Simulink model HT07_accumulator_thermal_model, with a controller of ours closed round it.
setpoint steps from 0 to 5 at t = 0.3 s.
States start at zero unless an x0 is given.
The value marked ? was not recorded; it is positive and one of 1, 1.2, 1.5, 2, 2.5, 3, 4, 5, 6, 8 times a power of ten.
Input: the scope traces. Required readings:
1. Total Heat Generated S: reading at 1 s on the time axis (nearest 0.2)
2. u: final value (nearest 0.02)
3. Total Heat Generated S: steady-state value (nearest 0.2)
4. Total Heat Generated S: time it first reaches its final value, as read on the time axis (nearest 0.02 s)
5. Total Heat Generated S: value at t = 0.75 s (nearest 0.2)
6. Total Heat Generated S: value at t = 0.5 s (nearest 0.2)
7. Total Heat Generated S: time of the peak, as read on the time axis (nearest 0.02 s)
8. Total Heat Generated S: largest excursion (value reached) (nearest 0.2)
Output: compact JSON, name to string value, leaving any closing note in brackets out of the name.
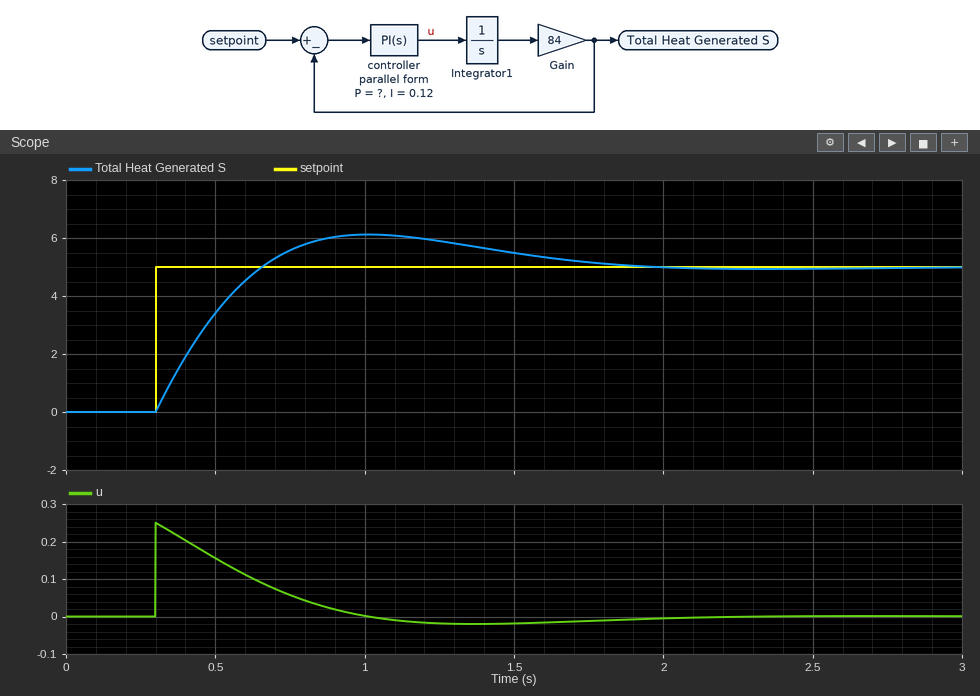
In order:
{"Total Heat Generated S: reading at 1 s on the time axis": "6.2", "u: final value": "0.00", "Total Heat Generated S: steady-state value": "5.0", "Total Heat Generated S: time it first reaches its final value, as read on the time axis": "0.66 s", "Total Heat Generated S: value at t = 0.75 s": "5.6", "Total Heat Generated S: value at t = 0.5 s": "3.4", "Total Heat Generated S: time of the peak, as read on the time axis": "1.02 s", "Total Heat Generated S: largest excursion (value reached)": "6.2"}
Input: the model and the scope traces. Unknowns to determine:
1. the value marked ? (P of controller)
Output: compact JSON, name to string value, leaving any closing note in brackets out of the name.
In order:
{"the value marked ?": "0.05"}
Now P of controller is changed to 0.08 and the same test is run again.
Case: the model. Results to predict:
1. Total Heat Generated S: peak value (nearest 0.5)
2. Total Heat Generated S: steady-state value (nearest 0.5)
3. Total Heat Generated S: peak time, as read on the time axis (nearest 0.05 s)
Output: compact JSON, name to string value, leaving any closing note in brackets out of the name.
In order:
{"Total Heat Generated S: peak value": "5.5", "Total Heat Generated S: steady-state value": "5.0", "Total Heat Generated S: peak time, as read on the time axis": "0.90 s"}
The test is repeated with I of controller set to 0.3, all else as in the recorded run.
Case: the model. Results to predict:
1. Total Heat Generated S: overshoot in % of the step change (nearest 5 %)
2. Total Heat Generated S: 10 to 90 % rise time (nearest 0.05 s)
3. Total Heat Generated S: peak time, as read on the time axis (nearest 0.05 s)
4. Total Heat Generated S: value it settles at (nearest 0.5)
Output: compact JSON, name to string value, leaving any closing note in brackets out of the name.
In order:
{"Total Heat Generated S: overshoot in % of the step change": "35 %", "Total Heat Generated S: 10 to 90 % rise time": "0.20 s", "Total Heat Generated S: peak time, as read on the time axis": "0.80 s", "Total Heat Generated S: value it settles at": "5.0"}
